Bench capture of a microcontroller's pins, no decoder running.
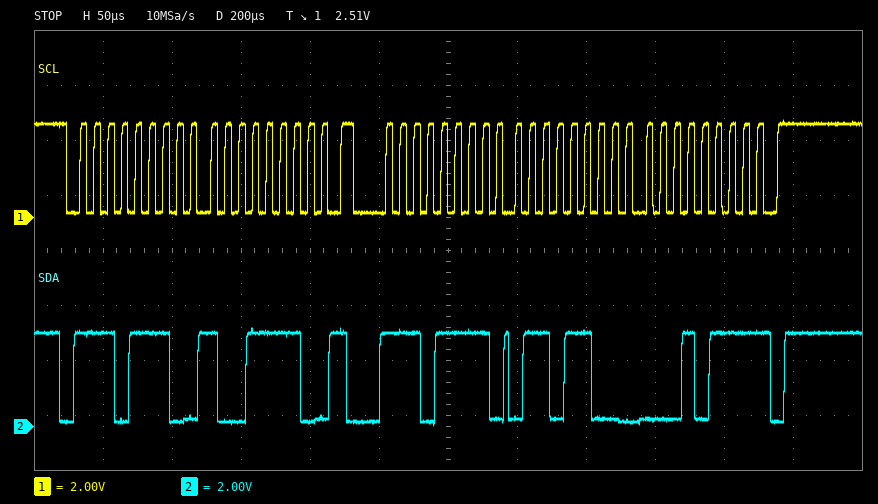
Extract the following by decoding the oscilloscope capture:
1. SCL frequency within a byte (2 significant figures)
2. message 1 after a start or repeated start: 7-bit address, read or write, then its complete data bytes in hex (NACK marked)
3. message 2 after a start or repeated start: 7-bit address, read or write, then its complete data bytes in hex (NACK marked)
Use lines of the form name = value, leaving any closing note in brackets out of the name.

SCL frequency within a byte = 100 kHz
message 1 after a start or repeated start: 7-bit address, read or write, then its complete data bytes in hex = 0x77 write: 9E
message 2 after a start or repeated start: 7-bit address, read or write, then its complete data bytes in hex = 0x77 read: 6C 17 NACK
